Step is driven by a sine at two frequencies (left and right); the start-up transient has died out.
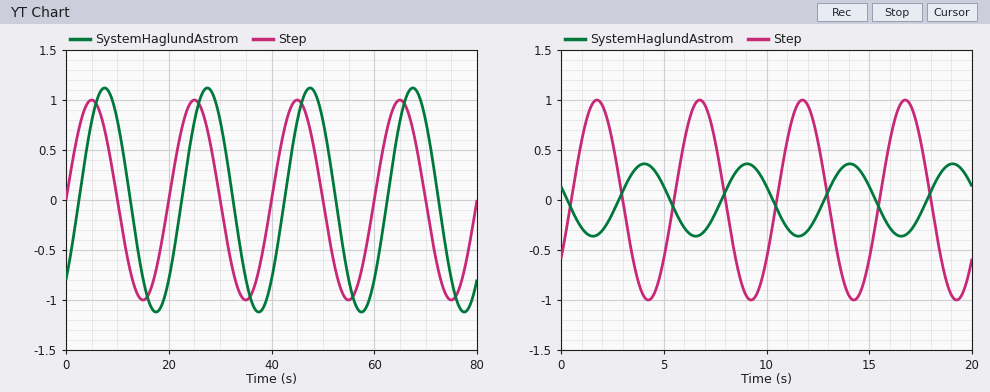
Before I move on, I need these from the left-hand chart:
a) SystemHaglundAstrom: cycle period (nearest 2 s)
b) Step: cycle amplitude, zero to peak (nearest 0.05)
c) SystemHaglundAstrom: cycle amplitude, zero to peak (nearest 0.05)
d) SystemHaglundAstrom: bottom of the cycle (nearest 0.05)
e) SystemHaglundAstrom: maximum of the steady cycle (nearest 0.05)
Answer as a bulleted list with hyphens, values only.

- 20 s
- 1.00
- 1.10
- -1.10
- 1.10
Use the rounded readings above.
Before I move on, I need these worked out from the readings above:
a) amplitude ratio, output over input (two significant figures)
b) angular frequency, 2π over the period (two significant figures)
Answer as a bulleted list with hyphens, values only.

- 1.1
- 0.31 rad/s
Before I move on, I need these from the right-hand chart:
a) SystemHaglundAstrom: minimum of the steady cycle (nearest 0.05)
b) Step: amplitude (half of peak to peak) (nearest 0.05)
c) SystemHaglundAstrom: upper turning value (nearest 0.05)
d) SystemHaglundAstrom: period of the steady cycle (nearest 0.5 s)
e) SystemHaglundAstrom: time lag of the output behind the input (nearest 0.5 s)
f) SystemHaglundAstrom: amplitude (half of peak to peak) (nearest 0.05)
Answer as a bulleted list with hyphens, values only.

- -0.35
- 1.00
- 0.35
- 5.0 s
- 2.5 s
- 0.35
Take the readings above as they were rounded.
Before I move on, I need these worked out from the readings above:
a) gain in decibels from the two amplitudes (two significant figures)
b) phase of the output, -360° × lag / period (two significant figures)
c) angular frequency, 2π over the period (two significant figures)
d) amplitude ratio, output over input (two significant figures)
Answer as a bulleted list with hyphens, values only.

- -9.1 dB
- -180°
- 1.3 rad/s
- 0.35
